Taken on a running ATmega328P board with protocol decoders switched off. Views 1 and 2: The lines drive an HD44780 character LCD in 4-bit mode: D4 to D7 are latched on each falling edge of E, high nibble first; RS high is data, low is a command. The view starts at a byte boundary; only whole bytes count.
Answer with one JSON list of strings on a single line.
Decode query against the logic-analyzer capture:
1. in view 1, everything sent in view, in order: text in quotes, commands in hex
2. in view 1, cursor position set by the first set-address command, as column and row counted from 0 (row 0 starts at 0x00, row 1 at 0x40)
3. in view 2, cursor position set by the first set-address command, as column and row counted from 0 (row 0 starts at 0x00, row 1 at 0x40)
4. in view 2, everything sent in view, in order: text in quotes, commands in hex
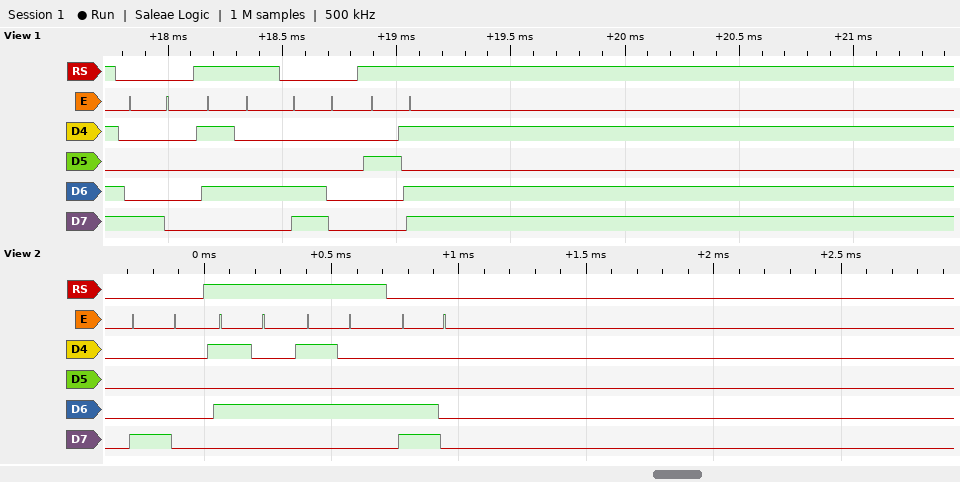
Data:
["0x80 \"T\" 0xC0 \"-\"", "column 0, row 0", "column 0, row 0", "0x80 \"TT\" 0xC0"]
